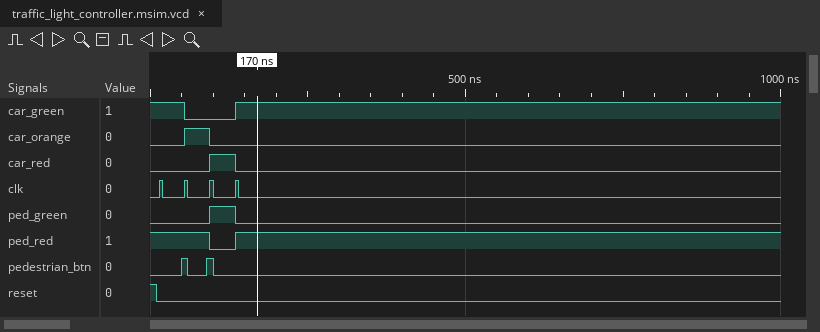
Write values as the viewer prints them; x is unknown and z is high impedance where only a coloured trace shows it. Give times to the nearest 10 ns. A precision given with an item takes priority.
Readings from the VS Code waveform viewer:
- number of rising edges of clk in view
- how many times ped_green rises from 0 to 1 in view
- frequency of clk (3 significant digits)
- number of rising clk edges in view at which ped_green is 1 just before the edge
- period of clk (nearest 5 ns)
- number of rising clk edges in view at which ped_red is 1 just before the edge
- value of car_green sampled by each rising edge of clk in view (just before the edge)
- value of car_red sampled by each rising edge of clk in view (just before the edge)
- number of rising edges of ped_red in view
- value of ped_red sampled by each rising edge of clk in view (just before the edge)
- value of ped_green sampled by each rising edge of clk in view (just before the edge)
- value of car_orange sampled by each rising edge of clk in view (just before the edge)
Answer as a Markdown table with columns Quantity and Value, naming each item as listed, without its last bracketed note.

| Quantity | Value |
|---|---|
| number of rising edges of clk in view | 4 |
| how many times ped_green rises from 0 to 1 in view | 1 |
| frequency of clk | 25.0 MHz |
| number of rising clk edges in view at which ped_green is 1 just before the edge | 1 |
| period of clk | 40 ns |
| number of rising clk edges in view at which ped_red is 1 just before the edge | 3 |
| value of car_green sampled by each rising edge of clk in view | 1 1 0 0 |
| value of car_red sampled by each rising edge of clk in view | 0 0 0 1 |
| number of rising edges of ped_red in view | 1 |
| value of ped_red sampled by each rising edge of clk in view | 1 1 1 0 |
| value of ped_green sampled by each rising edge of clk in view | 0 0 0 1 |
| value of car_orange sampled by each rising edge of clk in view | 0 0 1 0 |
